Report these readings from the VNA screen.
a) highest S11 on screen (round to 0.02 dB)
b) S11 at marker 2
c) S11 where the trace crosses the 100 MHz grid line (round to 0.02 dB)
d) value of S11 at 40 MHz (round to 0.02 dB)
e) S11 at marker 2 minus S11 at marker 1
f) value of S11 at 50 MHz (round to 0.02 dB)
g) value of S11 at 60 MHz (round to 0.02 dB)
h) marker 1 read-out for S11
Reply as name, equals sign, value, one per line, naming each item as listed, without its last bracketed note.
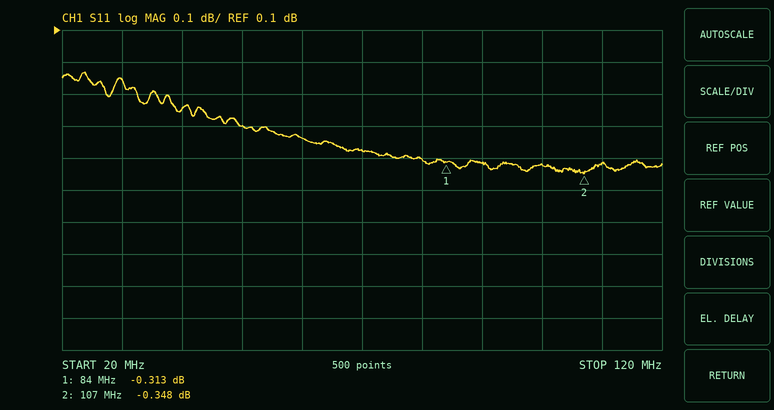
highest S11 on screen = -0.04 dB
S11 at marker 2 = -0.348 dB
S11 where the trace crosses the 100 MHz grid line = -0.32 dB
value of S11 at 40 MHz = -0.14 dB
S11 at marker 2 minus S11 at marker 1 = -0.035 dB
value of S11 at 50 MHz = -0.20 dB
value of S11 at 60 MHz = -0.24 dB
marker 1 read-out for S11 = -0.313 dB
